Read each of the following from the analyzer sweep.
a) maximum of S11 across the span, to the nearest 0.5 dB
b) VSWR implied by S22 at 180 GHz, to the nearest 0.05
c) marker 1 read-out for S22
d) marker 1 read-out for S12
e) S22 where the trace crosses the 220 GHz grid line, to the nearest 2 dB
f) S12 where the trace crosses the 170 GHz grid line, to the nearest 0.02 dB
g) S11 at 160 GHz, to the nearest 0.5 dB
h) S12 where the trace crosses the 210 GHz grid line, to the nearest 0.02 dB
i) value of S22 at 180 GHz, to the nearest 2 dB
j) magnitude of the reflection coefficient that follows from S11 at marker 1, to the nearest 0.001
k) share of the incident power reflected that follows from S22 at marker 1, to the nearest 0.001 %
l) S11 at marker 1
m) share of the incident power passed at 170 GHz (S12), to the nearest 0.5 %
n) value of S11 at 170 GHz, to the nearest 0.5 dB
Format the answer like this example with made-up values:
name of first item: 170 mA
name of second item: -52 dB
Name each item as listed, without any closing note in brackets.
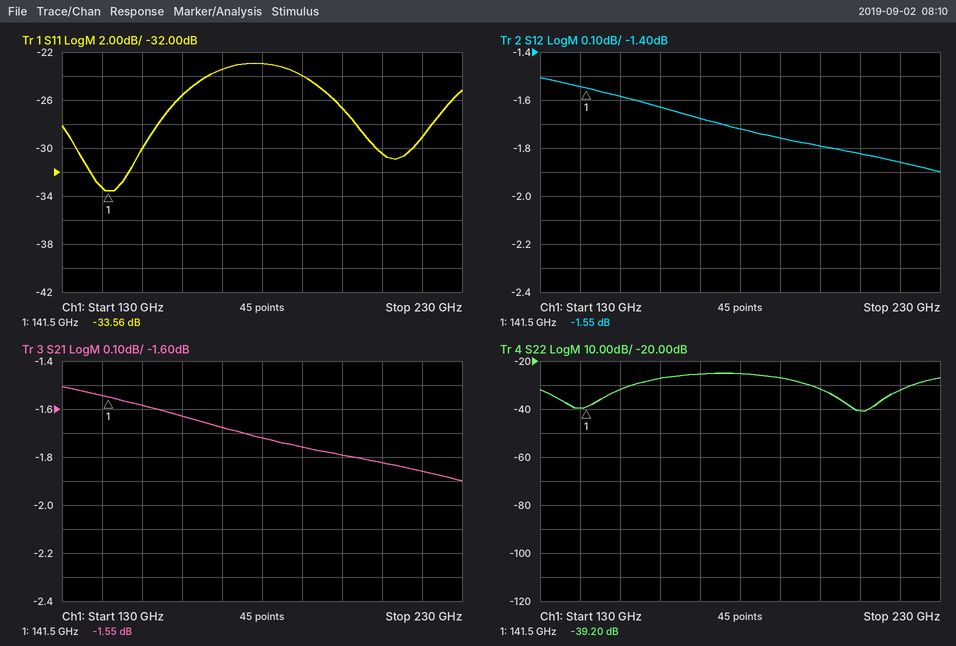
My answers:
maximum of S11 across the span, to the nearest 0.5 dB: -23.0 dB
VSWR implied by S22 at 180 GHz, to the nearest 0.05: 1.10
marker 1 read-out for S22: -39.20 dB
marker 1 read-out for S12: -1.55 dB
S22 where the trace crosses the 220 GHz grid line, to the nearest 2 dB: -32 dB
S12 where the trace crosses the 170 GHz grid line, to the nearest 0.02 dB: -1.68 dB
S11 at 160 GHz, to the nearest 0.5 dB: -25.5 dB
S12 where the trace crosses the 210 GHz grid line, to the nearest 0.02 dB: -1.82 dB
value of S22 at 180 GHz, to the nearest 2 dB: -26 dB
magnitude of the reflection coefficient that follows from S11 at marker 1, to the nearest 0.001: 0.021
share of the incident power reflected that follows from S22 at marker 1, to the nearest 0.001 %: 0.012 %
S11 at marker 1: -33.56 dB
share of the incident power passed at 170 GHz (S12), to the nearest 0.5 %: 68.0 %
value of S11 at 170 GHz, to the nearest 0.5 dB: -23.5 dB
